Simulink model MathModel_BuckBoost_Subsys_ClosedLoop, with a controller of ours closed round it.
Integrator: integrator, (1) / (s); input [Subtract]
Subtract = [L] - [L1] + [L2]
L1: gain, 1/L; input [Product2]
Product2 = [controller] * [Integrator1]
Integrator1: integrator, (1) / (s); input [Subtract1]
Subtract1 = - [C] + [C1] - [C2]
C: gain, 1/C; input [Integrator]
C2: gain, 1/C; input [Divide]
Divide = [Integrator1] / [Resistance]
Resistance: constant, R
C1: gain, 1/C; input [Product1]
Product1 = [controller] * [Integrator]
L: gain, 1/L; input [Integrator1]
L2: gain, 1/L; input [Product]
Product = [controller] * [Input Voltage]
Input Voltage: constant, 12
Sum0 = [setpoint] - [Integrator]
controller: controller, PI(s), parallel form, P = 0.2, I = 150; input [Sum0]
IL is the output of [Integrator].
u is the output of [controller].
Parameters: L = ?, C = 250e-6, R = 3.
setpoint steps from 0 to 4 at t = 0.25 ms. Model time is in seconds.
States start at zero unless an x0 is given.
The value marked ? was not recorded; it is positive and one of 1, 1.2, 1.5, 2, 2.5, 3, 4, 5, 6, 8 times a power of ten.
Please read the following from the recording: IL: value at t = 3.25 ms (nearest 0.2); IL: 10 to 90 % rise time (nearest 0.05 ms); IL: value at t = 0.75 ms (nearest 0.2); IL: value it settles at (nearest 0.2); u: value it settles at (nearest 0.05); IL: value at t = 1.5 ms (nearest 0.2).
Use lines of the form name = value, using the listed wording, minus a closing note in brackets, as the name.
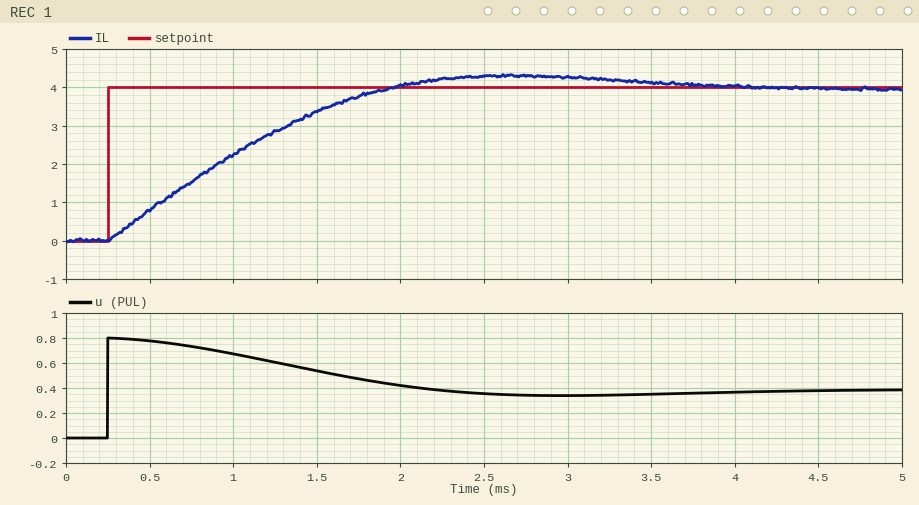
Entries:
IL: value at t = 3.25 ms = 4.2
IL: 10 to 90 % rise time = 1.25 ms
IL: value at t = 0.75 ms = 1.6
IL: value it settles at = 4.0
u: value it settles at = 0.40
IL: value at t = 1.5 ms = 3.4
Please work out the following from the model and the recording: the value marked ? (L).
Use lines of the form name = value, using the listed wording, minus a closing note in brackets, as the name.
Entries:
the value marked ? = 0.003
